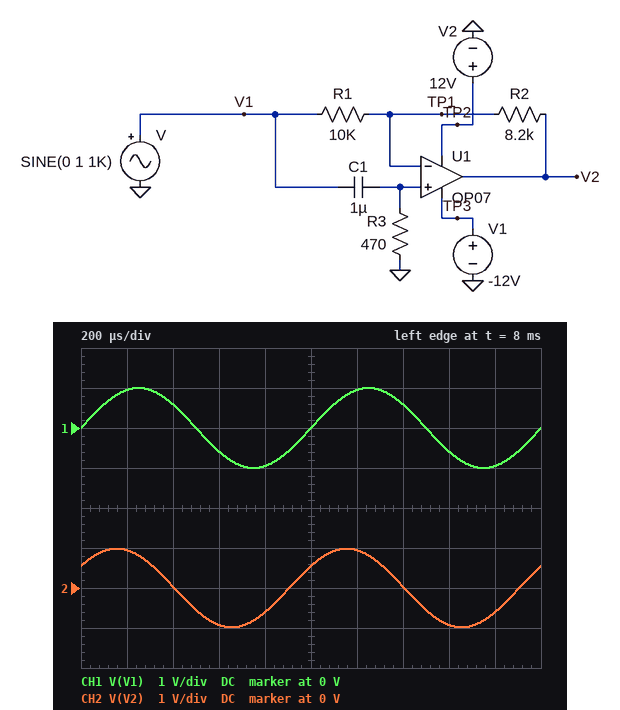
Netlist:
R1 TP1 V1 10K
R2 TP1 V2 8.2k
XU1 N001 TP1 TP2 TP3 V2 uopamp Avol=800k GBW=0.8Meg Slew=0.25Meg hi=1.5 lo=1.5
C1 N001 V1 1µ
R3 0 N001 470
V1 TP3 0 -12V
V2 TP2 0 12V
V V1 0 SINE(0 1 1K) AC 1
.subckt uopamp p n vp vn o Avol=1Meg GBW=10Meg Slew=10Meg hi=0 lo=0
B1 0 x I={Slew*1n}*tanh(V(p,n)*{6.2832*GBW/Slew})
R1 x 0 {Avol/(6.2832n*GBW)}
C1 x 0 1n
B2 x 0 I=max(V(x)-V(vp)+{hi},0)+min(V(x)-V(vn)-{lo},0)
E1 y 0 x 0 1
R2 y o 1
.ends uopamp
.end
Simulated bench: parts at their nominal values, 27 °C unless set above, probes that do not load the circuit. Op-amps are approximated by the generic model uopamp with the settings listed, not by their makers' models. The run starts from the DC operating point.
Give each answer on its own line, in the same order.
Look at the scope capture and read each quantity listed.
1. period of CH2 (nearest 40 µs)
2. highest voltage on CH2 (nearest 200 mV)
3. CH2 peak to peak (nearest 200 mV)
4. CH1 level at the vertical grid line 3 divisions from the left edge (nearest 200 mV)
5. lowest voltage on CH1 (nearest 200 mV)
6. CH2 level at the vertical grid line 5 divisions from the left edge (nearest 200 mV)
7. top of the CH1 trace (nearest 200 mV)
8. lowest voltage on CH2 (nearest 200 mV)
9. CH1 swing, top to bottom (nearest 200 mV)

1.00 ms
1.0 V
2.0 V
-600 mV
-1.0 V
600 mV
1.0 V
-1.0 V
2.0 V
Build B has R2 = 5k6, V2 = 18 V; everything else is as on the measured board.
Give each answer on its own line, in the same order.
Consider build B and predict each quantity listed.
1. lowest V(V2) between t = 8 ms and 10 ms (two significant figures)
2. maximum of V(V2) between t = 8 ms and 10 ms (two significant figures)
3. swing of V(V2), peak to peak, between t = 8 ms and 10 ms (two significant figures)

-960 mV
960 mV
1.9 V
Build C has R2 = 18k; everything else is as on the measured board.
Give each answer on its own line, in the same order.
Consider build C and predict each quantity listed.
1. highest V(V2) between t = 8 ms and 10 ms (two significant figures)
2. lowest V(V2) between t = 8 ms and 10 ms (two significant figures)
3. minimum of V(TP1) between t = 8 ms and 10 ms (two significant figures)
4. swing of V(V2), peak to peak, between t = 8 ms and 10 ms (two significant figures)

1.1 V
-1.1 V
-950 mV
2.2 V
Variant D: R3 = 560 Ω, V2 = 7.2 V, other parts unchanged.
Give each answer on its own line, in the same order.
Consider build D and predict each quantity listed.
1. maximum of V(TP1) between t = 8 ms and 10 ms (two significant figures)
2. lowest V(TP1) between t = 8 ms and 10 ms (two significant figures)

960 mV
-960 mV
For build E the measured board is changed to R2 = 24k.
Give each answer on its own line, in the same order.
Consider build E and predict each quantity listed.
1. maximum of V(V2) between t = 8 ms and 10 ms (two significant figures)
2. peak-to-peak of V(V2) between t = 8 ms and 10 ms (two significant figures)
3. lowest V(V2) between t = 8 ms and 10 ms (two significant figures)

1.2 V
2.4 V
-1.2 V
